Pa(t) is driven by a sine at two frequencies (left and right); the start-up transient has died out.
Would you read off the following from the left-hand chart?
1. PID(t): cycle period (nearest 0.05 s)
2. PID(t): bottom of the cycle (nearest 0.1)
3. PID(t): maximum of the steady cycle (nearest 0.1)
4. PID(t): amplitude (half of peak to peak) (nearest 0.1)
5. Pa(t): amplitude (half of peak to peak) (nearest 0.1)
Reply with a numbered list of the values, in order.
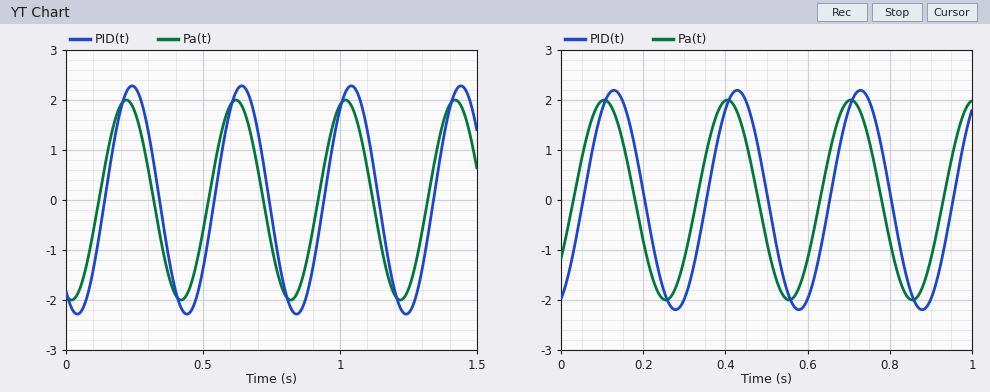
1. 0.40 s
2. -2.3
3. 2.3
4. 2.3
5. 2.0
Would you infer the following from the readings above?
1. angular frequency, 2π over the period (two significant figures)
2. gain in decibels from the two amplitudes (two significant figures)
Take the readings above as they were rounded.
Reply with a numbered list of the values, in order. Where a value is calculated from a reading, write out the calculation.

1. 2π / 0.4 = 16 rad/s
2. 20 log10(2.3 / 2) = 1.2 dB
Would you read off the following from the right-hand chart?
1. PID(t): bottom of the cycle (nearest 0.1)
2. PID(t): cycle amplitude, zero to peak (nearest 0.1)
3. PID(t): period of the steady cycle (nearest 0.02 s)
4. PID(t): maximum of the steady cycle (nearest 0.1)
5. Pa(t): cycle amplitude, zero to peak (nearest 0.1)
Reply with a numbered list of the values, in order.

1. -2.2
2. 2.2
3. 0.30 s
4. 2.2
5. 2.0
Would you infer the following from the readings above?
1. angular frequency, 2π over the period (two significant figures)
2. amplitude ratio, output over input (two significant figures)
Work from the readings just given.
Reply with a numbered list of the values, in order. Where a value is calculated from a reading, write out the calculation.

1. 2π / 0.3 = 21 rad/s
2. 2.2 / 2 = 1.1
